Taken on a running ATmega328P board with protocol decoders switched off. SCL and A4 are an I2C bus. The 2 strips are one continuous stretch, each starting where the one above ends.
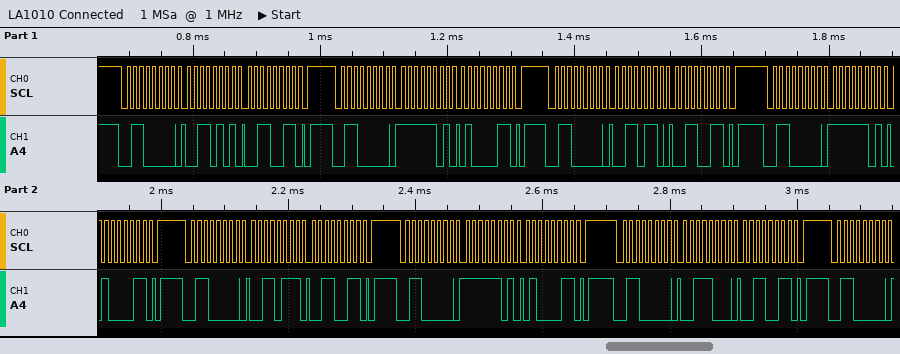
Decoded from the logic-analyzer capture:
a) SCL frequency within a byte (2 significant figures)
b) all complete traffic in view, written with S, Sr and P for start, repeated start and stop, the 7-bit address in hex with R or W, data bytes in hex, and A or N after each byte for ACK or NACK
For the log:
100 kHz
S 30W A 35 A 33 A P S 30W A FD A 43 A P S 30W A 36 A 33 A P S 30W A FD A 43 A P S 30W A 37 A 33 A P S 30W A FD A 43 A P S 30W A 38 A 33 A P S 30W A
